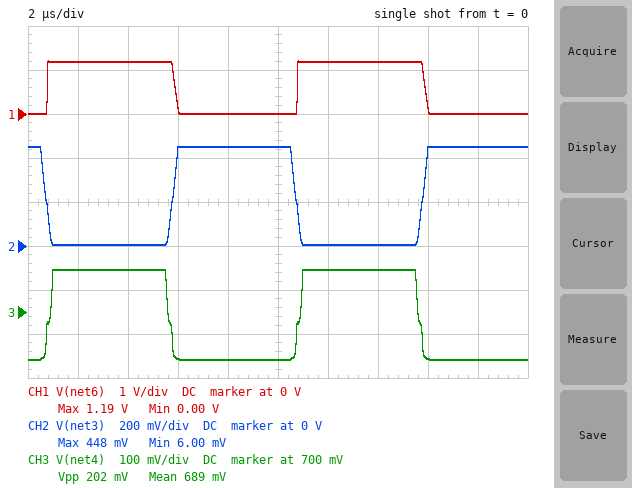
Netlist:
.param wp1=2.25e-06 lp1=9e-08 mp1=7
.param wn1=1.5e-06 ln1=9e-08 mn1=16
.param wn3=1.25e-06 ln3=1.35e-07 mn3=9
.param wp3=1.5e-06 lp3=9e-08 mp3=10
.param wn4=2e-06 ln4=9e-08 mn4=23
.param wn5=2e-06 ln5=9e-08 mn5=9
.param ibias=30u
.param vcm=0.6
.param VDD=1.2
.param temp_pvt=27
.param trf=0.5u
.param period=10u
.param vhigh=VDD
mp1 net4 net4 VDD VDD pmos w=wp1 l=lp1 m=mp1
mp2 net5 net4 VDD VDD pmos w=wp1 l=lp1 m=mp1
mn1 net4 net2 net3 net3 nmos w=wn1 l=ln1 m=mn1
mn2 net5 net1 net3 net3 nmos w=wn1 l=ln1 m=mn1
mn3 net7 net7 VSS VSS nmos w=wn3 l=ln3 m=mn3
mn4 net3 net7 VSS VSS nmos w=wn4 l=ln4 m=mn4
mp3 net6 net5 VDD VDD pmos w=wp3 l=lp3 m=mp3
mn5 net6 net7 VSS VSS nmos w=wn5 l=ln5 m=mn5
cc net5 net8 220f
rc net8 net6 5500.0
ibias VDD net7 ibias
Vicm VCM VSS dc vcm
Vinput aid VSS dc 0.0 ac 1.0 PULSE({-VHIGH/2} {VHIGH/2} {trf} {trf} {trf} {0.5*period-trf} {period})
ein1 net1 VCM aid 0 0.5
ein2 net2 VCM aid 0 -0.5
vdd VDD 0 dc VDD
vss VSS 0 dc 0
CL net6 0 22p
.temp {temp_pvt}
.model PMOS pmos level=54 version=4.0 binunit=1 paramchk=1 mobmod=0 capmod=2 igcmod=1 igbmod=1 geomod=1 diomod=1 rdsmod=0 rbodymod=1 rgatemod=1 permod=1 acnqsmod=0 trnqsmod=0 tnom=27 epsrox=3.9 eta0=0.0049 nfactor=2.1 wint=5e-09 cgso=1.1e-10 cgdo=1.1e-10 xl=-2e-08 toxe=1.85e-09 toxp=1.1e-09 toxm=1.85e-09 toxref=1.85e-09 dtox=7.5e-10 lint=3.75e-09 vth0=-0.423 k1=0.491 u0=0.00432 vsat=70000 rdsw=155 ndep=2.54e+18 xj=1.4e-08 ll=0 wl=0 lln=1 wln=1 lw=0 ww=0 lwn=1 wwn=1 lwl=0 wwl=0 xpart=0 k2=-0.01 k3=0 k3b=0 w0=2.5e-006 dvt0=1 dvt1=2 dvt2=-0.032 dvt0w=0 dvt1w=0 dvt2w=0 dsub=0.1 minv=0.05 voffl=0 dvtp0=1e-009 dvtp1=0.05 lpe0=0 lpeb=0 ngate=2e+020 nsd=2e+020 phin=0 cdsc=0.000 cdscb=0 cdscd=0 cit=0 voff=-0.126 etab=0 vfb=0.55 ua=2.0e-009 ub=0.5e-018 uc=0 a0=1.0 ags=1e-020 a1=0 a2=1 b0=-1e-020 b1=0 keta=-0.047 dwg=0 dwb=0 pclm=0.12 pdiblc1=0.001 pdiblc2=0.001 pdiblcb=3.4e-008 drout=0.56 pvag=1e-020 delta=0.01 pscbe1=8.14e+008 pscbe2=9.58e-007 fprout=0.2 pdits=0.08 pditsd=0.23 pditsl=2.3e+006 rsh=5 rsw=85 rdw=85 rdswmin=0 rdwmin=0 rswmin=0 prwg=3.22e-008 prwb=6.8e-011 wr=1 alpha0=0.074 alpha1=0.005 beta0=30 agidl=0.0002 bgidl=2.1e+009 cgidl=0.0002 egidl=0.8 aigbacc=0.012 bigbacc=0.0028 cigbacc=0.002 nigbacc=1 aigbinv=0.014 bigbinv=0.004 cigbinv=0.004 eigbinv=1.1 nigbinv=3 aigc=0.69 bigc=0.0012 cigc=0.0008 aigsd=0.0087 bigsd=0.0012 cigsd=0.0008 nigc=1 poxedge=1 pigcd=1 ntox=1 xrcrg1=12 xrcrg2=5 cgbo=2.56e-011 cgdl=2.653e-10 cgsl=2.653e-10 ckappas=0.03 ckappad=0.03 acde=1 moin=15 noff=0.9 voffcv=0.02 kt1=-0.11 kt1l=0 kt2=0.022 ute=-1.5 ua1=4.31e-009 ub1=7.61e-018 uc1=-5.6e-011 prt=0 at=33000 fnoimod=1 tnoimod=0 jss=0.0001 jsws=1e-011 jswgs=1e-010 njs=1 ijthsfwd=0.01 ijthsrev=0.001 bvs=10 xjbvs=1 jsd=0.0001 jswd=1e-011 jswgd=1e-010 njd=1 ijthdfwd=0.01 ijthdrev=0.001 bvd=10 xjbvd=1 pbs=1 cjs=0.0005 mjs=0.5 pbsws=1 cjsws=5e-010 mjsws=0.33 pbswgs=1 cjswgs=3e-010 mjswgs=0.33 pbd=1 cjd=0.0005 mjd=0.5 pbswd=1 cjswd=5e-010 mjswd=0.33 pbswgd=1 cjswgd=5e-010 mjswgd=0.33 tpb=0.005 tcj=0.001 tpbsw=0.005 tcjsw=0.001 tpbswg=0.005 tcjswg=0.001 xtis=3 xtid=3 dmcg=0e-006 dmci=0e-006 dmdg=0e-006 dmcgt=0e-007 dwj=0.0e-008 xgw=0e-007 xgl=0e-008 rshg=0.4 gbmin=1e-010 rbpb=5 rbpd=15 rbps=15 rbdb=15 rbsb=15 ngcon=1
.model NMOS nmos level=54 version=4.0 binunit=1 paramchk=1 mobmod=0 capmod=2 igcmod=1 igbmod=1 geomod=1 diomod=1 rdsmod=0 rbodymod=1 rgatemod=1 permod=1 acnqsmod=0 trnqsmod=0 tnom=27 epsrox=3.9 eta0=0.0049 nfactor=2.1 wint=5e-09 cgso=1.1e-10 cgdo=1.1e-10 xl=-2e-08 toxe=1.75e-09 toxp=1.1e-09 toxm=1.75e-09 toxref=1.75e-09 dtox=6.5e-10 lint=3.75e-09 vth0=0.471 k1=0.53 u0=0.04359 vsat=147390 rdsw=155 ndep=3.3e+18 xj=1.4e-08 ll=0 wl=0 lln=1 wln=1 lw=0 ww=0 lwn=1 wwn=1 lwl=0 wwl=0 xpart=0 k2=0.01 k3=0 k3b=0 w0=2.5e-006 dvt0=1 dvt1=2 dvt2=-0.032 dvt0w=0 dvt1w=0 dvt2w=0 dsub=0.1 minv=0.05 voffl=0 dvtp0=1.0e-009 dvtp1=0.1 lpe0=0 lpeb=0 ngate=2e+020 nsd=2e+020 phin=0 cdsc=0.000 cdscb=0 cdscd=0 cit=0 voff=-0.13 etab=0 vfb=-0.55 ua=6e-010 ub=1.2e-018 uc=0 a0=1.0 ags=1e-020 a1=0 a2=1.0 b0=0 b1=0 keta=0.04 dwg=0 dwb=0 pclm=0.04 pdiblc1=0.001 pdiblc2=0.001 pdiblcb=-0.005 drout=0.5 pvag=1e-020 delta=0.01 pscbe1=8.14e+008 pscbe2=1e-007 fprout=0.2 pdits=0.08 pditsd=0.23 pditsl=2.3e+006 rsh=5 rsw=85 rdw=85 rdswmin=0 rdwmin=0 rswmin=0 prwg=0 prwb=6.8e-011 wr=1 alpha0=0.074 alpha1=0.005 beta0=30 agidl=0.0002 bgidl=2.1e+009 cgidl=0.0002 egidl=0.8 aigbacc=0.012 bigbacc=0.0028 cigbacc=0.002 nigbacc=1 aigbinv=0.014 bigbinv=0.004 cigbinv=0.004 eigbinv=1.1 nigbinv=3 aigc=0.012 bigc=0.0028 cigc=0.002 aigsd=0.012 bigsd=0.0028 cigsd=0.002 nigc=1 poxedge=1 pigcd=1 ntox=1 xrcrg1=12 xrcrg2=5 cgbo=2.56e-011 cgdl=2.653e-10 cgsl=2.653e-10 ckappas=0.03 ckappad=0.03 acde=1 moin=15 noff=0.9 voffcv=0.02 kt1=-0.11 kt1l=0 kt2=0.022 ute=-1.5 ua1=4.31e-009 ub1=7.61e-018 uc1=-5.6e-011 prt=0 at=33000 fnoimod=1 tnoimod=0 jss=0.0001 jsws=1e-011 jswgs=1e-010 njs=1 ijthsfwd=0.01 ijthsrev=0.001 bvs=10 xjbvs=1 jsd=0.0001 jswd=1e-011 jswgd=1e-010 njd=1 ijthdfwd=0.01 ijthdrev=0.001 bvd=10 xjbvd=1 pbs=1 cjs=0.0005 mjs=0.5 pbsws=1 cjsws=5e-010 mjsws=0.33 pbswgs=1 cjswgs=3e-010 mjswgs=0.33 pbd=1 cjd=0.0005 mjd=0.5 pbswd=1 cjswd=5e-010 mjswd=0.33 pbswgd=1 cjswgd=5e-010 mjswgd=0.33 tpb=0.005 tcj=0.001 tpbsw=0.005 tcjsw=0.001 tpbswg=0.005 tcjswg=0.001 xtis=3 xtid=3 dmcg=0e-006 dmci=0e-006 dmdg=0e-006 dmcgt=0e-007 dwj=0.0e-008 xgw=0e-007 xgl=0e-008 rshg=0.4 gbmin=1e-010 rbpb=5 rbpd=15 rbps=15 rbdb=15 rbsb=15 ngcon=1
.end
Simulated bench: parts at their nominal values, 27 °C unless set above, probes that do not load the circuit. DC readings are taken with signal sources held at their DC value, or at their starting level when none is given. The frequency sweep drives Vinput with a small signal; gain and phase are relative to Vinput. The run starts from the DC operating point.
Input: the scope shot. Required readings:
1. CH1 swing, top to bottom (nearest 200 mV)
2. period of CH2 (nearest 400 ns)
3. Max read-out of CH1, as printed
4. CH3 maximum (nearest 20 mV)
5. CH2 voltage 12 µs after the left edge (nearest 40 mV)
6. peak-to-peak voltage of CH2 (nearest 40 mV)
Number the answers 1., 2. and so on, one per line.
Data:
1. 1.2 V
2. 10.0 µs
3. 1.19 V
4. 800 mV
5. 0 V
6. 440 mV
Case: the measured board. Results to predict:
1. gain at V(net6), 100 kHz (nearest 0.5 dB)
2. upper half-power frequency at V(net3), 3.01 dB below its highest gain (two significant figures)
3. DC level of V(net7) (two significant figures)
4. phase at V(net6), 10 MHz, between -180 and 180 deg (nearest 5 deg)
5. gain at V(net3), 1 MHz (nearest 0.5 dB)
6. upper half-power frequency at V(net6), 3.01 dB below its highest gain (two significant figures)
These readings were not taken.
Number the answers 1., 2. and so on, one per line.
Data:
1. 56.0 dB
2. 25 MHz
3. 410 mV
4. -100 deg
5. -13.0 dB
6. 350 kHz
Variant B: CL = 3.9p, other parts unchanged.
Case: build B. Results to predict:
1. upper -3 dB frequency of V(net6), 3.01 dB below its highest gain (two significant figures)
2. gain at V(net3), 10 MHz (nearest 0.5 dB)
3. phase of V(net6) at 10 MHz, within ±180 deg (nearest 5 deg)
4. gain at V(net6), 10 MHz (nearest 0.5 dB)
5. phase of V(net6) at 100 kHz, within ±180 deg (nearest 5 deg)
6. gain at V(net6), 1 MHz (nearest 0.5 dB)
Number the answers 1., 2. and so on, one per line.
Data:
1. 1.1 MHz
2. -16.0 dB
3. -90 deg
4. 36.5 dB
5. -5 deg
6. 53.5 dB
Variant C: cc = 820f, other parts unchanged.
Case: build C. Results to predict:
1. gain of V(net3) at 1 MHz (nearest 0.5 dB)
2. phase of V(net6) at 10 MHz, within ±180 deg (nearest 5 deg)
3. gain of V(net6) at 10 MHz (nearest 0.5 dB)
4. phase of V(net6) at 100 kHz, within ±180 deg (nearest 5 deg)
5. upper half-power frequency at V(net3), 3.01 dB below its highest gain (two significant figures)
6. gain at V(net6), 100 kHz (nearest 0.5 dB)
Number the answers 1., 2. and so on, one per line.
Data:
1. -16.0 dB
2. -110 deg
3. 22.5 dB
4. -25 deg
5. 430 kHz
6. 55.5 dB
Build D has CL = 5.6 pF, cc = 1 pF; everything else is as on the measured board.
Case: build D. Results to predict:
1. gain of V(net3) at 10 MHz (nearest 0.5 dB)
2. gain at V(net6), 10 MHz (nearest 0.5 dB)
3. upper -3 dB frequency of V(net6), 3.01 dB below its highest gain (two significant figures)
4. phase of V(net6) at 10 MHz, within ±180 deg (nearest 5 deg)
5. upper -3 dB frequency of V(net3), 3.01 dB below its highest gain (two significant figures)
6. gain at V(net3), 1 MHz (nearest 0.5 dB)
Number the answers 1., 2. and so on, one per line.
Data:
1. -23.0 dB
2. 27.0 dB
3. 340 kHz
4. -90 deg
5. 370 kHz
6. -19.5 dB
